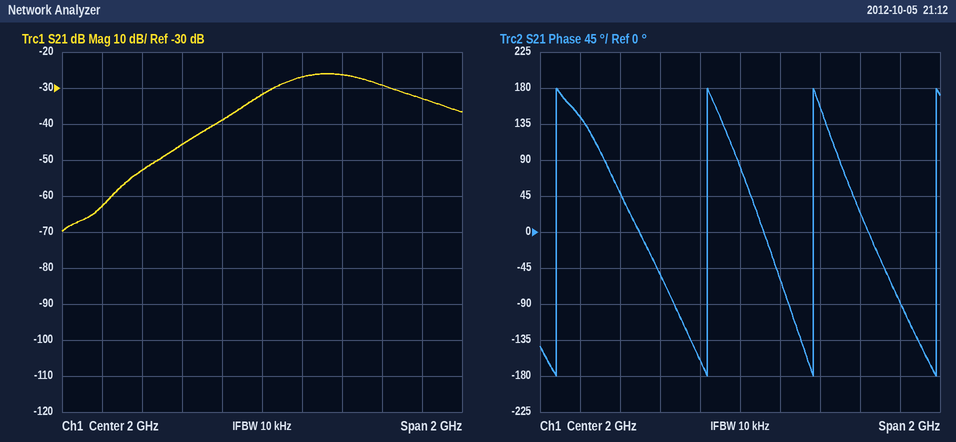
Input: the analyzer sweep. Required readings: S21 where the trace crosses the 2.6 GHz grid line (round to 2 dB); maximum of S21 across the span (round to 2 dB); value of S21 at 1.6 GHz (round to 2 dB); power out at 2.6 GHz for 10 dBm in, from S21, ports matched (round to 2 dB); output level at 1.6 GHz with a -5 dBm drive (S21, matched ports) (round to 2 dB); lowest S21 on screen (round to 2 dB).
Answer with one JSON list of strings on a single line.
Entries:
["-30 dB", "-26 dB", "-46 dB", "-20 dBm", "-50 dBm", "-70 dB"]
